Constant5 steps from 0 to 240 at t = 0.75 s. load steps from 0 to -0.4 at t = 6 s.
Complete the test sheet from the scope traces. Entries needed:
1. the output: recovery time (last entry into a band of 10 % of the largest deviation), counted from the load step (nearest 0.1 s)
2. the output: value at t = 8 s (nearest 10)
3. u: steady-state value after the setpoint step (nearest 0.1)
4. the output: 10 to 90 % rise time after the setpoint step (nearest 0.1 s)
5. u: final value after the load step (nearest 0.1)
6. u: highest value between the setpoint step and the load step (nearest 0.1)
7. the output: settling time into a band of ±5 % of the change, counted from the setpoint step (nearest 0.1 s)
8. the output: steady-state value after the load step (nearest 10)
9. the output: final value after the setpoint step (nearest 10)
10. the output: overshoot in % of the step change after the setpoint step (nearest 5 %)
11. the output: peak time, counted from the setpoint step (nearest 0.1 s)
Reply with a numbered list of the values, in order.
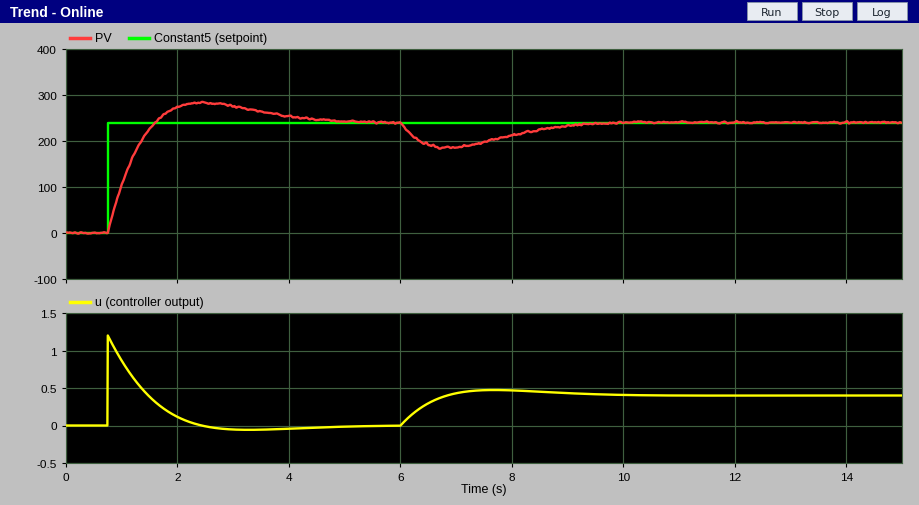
1. 3.2 s
2. 210
3. 0.0
4. 0.6 s
5. 0.4
6. 1.2
7. 3.4 s
8. 240
9. 240
10. 20 %
11. 1.7 s
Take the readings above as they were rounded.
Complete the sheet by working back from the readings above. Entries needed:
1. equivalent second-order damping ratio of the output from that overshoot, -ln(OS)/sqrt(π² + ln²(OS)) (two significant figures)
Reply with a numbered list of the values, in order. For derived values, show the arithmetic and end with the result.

1. ln(0.2) = -1.609; 1.609 / sqrt(9.870 + 2.590) = 0.46
